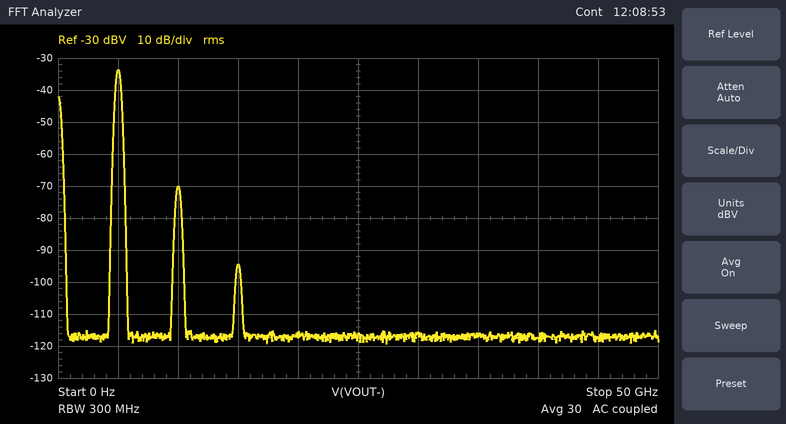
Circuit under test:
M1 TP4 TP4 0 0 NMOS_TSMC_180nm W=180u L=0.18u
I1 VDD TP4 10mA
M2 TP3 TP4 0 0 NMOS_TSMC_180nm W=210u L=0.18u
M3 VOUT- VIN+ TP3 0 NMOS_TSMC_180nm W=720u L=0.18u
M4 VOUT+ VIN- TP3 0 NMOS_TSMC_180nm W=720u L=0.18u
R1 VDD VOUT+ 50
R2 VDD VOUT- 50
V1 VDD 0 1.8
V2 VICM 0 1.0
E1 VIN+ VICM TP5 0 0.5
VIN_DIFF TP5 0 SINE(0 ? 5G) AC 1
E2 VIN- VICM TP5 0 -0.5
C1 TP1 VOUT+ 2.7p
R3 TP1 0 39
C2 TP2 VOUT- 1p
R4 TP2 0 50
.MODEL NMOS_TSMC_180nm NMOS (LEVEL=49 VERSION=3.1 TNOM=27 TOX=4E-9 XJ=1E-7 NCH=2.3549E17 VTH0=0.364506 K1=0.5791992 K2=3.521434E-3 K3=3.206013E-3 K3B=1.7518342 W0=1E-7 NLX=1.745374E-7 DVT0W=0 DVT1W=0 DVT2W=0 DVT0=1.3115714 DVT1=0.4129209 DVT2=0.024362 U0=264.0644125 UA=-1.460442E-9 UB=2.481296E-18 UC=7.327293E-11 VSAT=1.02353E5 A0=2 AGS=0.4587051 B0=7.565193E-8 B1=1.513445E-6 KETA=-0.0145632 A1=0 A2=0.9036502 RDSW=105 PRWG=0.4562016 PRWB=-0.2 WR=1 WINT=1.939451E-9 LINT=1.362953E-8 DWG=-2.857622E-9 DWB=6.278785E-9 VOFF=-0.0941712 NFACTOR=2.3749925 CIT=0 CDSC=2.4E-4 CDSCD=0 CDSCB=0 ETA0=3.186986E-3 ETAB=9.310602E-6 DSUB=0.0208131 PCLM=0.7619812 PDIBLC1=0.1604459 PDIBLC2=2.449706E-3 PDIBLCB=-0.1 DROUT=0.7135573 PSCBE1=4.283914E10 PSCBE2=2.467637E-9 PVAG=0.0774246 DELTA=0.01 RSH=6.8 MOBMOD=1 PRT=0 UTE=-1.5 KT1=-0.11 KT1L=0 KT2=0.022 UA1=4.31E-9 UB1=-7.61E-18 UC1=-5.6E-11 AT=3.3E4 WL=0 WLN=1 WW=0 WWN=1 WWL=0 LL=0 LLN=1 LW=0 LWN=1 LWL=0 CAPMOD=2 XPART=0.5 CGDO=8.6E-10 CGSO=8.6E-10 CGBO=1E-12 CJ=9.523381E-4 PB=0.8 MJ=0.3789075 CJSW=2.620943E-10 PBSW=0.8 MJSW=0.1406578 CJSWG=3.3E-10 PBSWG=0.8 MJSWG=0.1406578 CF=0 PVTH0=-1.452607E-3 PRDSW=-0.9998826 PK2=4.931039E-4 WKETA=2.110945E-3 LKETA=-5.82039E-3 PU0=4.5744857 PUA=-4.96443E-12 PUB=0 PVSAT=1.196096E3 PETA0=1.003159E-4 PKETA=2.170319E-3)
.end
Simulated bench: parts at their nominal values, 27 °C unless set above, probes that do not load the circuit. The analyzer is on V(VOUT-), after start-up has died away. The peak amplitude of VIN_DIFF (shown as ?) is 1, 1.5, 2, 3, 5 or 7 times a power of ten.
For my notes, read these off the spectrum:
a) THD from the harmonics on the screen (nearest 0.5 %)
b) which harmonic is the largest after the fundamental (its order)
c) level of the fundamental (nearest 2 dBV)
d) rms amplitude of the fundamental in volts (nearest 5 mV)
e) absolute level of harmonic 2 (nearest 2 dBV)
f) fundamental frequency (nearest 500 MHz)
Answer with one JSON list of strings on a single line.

["1.5 %", "2", "-34 dBV", "20 mV", "-70 dBV", "5.0 GHz"]
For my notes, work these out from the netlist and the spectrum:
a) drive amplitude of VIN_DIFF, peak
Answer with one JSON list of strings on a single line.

["50 mV"]
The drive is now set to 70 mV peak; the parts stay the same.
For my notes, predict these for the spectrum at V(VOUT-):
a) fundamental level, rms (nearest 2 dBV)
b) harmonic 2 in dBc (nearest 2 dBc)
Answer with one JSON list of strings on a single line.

["-30 dBV", "-34 dBc"]
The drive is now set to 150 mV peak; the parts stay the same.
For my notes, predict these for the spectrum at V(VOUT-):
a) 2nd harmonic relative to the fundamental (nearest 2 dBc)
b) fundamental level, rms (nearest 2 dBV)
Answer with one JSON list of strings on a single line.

["-26 dBc", "-24 dBV"]
